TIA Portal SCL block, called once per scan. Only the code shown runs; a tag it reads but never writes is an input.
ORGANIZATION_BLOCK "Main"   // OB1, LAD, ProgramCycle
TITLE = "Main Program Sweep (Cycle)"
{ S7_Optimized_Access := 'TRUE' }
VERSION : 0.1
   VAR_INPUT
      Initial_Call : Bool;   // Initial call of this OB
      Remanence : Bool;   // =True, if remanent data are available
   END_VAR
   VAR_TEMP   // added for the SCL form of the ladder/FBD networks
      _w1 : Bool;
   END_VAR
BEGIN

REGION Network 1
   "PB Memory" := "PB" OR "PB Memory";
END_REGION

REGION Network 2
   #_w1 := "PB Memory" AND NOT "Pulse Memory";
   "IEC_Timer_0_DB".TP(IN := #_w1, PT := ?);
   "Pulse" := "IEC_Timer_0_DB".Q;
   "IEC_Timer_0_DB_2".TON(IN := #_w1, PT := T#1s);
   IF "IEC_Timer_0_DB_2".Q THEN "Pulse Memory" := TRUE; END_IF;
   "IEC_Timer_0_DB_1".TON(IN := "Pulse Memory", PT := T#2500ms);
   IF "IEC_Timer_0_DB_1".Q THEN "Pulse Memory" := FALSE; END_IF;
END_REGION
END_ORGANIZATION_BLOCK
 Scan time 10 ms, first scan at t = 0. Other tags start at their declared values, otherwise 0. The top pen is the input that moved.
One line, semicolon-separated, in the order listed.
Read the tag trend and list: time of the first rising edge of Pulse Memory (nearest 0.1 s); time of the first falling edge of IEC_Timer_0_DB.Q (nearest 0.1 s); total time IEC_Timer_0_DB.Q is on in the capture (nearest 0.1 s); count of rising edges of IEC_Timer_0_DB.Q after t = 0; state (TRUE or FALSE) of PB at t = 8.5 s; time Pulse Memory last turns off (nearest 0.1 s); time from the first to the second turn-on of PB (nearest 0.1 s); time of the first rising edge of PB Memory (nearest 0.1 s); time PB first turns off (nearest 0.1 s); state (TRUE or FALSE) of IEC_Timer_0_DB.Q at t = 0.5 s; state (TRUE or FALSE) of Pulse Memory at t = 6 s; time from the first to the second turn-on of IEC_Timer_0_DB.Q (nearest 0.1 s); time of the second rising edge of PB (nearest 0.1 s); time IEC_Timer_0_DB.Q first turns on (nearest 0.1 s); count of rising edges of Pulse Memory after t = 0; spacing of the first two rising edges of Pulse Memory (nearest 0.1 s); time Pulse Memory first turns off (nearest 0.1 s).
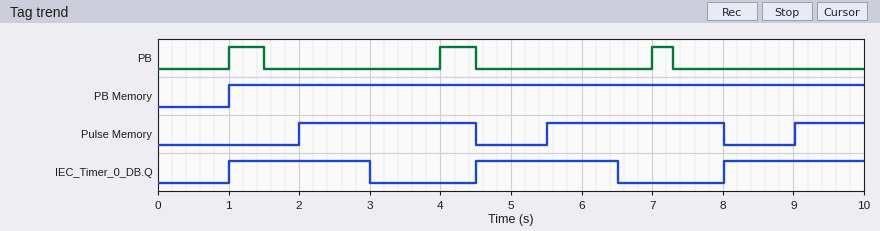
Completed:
2.0 s; 3.0 s; 6.0 s; 3; FALSE; 8.0 s; 3.0 s; 1.0 s; 1.5 s; FALSE; TRUE; 3.5 s; 4.0 s; 1.0 s; 3; 3.5 s; 4.5 s
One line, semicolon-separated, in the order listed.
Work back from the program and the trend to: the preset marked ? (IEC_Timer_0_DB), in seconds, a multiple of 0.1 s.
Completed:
2.0 s
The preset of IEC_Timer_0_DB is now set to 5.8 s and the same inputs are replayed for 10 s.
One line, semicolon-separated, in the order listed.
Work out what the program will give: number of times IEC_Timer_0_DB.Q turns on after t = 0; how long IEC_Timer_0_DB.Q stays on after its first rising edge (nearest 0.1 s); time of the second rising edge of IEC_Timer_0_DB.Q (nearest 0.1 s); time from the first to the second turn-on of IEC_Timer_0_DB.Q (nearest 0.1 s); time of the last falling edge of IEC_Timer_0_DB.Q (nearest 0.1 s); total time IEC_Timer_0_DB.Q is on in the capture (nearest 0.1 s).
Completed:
2; 5.8 s; 8.0 s; 7.0 s; 6.8 s; 7.8 s
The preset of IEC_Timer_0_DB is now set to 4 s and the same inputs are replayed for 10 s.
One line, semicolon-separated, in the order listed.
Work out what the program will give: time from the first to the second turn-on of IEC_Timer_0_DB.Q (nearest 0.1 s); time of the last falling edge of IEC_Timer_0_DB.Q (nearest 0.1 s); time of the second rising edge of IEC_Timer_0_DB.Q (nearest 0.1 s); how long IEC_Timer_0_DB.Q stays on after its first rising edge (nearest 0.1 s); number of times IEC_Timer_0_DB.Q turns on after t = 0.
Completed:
7.0 s; 5.0 s; 8.0 s; 4.0 s; 2
